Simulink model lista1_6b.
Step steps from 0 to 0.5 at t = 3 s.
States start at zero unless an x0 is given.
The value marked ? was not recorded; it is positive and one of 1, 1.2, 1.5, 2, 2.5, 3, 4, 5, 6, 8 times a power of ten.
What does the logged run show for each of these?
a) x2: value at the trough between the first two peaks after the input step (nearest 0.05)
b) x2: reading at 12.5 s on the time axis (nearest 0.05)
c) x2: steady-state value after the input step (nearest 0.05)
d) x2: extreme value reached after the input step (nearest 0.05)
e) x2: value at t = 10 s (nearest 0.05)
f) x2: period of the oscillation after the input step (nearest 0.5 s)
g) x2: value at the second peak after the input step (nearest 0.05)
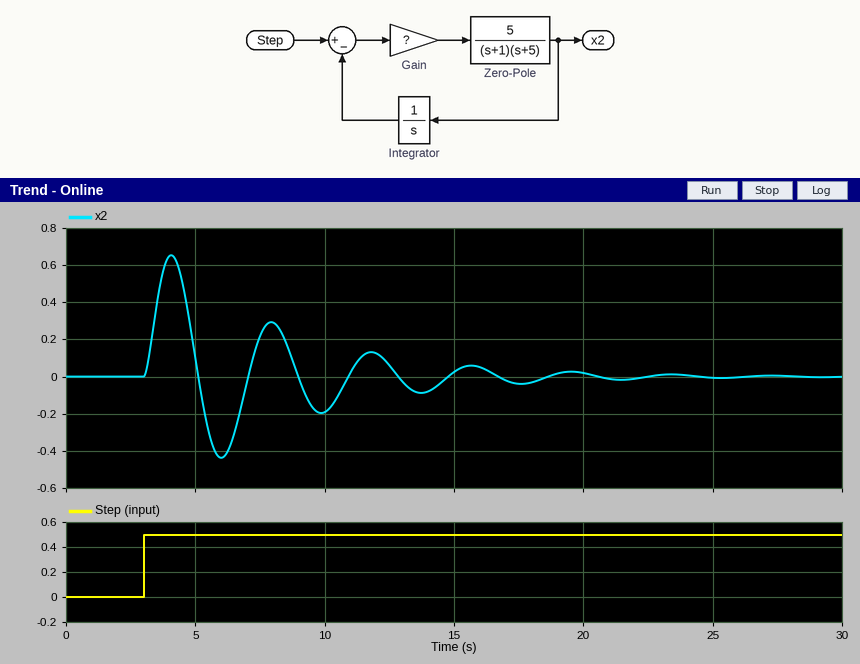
-0.45
0.05
0.00
0.65
-0.20
4.0 s
0.30
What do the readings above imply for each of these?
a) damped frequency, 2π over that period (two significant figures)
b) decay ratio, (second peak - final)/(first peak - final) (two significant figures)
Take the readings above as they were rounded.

1.6 rad/s
0.46
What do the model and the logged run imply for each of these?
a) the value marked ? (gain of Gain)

3
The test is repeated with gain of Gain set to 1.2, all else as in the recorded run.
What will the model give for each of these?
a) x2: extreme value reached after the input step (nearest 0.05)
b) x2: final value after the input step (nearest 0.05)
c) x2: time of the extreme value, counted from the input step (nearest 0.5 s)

0.35
0.00
1.5 s
